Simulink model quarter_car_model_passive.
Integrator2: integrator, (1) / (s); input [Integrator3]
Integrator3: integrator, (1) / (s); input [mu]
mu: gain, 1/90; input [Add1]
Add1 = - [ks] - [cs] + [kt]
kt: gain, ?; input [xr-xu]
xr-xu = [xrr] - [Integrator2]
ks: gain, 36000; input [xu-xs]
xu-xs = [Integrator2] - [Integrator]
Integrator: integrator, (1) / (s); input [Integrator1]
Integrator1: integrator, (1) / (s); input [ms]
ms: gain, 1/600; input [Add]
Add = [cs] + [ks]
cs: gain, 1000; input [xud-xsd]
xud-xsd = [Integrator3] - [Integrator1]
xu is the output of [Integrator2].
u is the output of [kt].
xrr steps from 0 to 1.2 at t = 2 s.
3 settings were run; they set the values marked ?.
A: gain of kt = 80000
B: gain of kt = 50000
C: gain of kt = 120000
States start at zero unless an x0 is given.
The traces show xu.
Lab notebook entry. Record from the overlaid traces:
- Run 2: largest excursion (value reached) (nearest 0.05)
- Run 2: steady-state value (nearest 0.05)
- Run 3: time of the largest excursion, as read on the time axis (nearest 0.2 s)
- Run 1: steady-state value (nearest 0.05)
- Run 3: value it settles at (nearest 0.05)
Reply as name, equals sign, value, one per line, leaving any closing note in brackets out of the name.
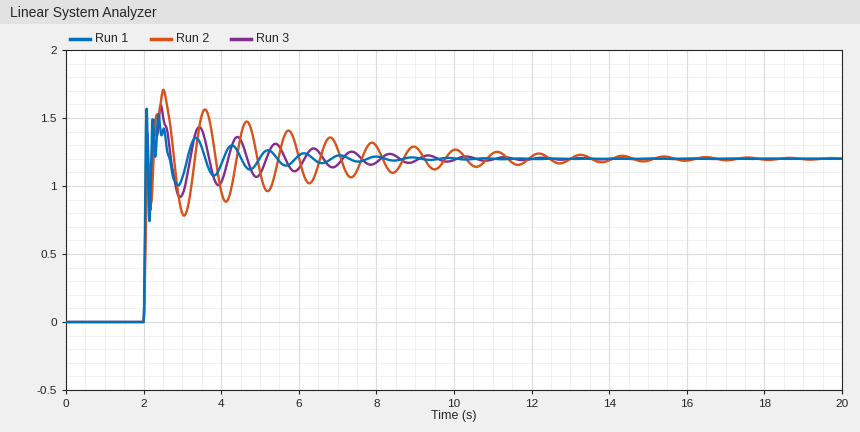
Run 2: largest excursion (value reached) = 1.70
Run 2: steady-state value = 1.20
Run 3: time of the largest excursion, as read on the time axis = 2.4 s
Run 1: steady-state value = 1.20
Run 3: value it settles at = 1.20
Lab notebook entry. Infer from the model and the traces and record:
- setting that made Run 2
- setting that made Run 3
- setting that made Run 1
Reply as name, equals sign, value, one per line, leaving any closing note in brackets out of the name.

setting that made Run 2 = B
setting that made Run 3 = A
setting that made Run 1 = C
